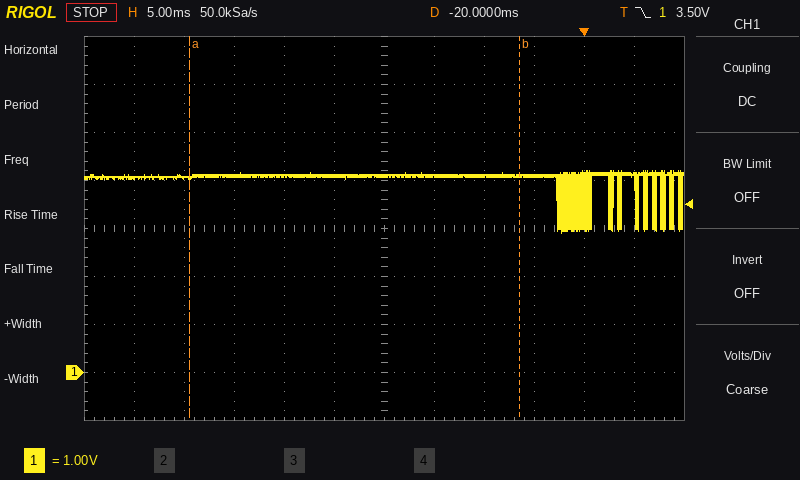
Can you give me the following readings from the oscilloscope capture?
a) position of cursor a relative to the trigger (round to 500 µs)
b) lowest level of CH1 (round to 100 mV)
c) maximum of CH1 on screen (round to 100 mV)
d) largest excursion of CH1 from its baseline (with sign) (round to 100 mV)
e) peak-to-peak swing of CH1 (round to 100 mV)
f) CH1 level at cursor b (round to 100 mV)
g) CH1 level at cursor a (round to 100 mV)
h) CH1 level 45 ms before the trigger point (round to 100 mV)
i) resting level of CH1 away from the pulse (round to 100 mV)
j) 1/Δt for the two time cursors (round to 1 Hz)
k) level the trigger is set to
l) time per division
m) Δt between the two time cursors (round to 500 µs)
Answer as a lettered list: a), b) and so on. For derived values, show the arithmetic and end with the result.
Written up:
a) -39.5 ms
b) 2.9 V
c) 4.2 V
d) 2.9 V − (4.1 V) = -1.2 V
e) 4.2 V − (2.9 V) = 1.3 V
f) 4.1 V
g) 4.1 V
h) 4.1 V
i) 4.1 V
j) 1 / 33.0 ms ≈ 30 Hz
k) 3.50 V
l) 5 ms
m) 33.0 ms
